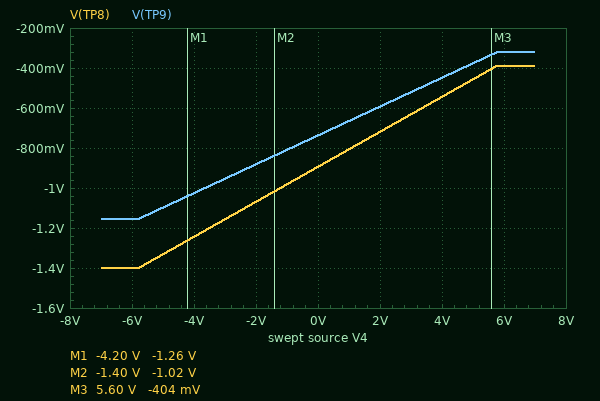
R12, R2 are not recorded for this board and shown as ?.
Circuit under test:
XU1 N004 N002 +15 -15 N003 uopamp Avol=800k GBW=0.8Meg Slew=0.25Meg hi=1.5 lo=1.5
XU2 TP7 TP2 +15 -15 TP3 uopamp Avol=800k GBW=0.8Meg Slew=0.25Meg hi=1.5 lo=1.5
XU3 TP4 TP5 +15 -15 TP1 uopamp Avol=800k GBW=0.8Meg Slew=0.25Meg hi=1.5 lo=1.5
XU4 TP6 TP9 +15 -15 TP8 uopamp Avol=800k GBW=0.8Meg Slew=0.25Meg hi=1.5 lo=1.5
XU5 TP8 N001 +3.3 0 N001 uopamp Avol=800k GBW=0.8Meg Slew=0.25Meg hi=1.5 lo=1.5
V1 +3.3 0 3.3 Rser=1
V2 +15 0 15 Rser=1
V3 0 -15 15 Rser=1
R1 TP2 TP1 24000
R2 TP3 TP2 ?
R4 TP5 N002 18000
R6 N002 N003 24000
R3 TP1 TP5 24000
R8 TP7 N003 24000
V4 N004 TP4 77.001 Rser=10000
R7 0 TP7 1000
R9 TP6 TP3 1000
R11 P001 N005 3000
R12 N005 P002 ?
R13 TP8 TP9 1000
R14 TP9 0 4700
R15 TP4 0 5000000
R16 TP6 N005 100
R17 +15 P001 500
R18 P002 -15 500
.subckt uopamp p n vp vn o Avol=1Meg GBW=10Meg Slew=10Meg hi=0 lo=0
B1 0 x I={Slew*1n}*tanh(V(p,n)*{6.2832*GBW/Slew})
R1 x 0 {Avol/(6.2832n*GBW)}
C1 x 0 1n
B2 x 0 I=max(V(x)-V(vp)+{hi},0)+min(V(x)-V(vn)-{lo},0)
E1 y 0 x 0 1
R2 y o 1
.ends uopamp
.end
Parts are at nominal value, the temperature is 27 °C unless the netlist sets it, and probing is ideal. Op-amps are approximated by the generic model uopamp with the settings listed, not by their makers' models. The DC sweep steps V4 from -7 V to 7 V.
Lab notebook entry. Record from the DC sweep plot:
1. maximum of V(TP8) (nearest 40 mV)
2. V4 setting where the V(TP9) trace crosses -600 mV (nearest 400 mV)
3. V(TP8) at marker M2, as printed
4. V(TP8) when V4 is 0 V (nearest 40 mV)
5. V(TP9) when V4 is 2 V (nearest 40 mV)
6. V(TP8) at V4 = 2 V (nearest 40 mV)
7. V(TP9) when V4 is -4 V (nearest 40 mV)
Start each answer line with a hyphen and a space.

- -400 mV
- 2.0 V
- -1.02 V
- -880 mV
- -600 mV
- -720 mV
- -1.04 V
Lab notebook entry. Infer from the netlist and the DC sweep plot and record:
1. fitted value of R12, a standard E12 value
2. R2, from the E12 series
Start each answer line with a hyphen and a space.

- 2.2 kΩ
- 390 Ω
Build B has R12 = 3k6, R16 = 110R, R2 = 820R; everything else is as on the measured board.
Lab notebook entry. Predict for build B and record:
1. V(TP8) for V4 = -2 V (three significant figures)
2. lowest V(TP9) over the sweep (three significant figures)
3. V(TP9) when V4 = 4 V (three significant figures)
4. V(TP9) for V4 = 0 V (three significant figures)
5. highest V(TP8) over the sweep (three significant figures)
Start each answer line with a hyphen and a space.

- 249 mV
- -153 mV
- 774 mV
- 395 mV
- 1.14 V
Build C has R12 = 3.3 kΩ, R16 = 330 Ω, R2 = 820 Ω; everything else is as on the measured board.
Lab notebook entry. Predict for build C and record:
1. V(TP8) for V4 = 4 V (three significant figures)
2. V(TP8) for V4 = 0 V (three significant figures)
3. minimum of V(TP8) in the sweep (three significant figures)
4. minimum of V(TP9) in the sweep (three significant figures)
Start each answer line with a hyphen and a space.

- 708 mV
- 237 mV
- -443 mV
- -366 mV
